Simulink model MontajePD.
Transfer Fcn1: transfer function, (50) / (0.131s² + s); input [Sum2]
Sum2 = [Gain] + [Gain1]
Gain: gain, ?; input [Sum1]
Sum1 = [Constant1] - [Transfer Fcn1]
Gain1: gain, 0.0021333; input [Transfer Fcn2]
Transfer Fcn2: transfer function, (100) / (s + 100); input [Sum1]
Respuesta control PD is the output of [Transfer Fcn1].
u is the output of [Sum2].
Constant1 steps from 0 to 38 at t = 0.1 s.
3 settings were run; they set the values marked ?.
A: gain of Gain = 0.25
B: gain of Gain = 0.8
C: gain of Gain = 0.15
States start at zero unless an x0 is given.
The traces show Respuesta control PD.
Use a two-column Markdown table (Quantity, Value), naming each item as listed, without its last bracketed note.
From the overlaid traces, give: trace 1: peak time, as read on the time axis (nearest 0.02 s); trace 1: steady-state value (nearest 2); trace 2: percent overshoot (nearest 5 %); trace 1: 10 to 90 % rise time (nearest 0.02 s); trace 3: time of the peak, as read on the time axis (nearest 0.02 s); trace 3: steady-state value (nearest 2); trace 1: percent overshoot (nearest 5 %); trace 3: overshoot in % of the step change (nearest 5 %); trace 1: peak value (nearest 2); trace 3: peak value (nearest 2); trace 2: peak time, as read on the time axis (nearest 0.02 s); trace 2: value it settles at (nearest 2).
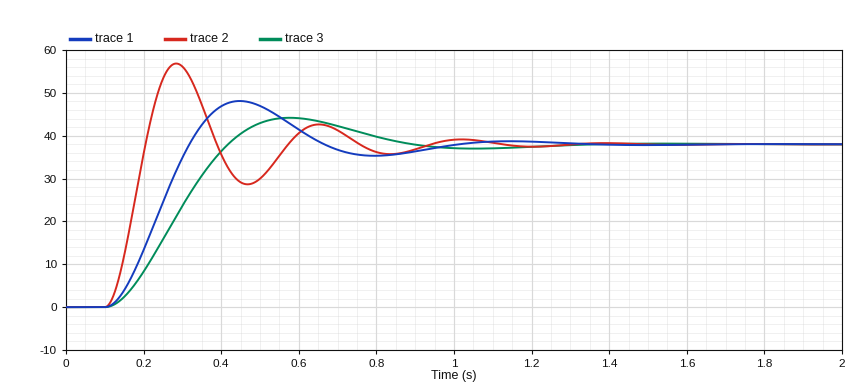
| Quantity | Value |
|---|---|
| trace 1: peak time, as read on the time axis | 0.44 s |
| trace 1: steady-state value | 38 |
| trace 2: percent overshoot | 50 % |
| trace 1: 10 to 90 % rise time | 0.14 s |
| trace 3: time of the peak, as read on the time axis | 0.58 s |
| trace 3: steady-state value | 38 |
| trace 1: percent overshoot | 25 % |
| trace 3: overshoot in % of the step change | 15 % |
| trace 1: peak value | 48 |
| trace 3: peak value | 44 |
| trace 2: peak time, as read on the time axis | 0.28 s |
| trace 2: value it settles at | 38 |
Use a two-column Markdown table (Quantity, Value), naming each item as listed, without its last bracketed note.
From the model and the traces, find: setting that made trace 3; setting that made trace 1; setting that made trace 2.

| Quantity | Value |
|---|---|
| setting that made trace 3 | C |
| setting that made trace 1 | A |
| setting that made trace 2 | B |
